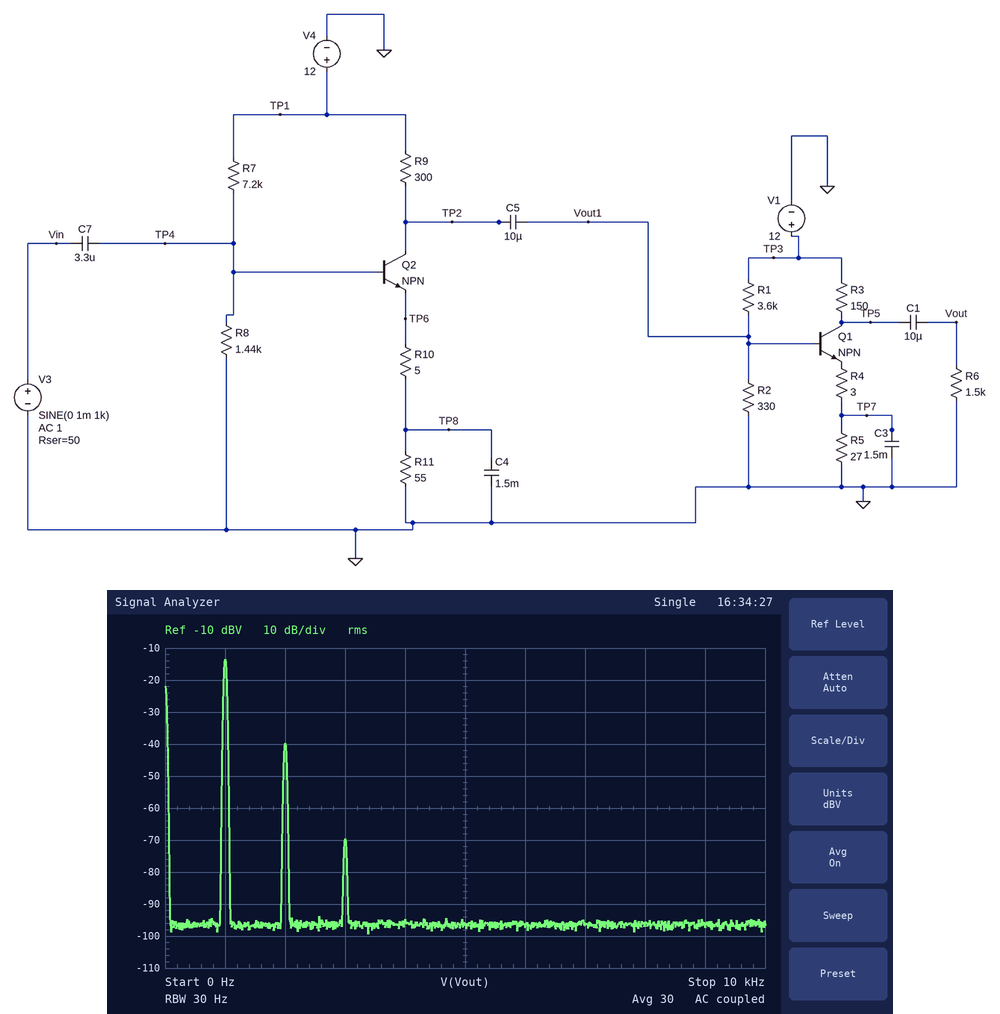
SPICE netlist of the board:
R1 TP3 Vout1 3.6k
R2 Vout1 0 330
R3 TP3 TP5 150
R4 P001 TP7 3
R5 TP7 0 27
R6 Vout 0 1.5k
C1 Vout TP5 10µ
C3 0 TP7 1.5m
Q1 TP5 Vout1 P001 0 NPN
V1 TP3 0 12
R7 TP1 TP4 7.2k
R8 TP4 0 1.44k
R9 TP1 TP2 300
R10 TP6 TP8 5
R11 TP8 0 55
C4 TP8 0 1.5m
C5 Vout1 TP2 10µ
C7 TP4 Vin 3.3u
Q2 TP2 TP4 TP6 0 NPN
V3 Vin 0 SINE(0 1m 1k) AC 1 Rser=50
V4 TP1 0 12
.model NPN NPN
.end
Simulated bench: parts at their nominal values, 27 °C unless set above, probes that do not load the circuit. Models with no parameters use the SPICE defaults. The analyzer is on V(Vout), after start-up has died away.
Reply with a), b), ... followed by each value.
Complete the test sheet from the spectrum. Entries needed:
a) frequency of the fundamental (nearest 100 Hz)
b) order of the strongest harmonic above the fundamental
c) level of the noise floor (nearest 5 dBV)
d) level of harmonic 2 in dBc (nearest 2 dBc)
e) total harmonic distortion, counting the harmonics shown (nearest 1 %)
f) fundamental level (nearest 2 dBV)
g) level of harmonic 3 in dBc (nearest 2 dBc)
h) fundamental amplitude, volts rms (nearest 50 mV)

a) 1.0 kHz
b) 2
c) -95 dBV
d) -26 dBc
e) 5 %
f) -14 dBV
g) -56 dBc
h) 200 mV
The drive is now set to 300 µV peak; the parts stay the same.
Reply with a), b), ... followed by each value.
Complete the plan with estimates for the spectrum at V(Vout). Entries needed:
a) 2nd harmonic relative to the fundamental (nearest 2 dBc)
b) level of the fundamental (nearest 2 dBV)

a) -36 dBc
b) -24 dBV
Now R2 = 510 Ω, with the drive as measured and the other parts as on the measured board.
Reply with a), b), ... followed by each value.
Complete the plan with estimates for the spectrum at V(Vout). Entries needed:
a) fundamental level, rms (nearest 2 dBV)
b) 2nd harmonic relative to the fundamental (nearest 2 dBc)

a) -8 dBV
b) -38 dBc
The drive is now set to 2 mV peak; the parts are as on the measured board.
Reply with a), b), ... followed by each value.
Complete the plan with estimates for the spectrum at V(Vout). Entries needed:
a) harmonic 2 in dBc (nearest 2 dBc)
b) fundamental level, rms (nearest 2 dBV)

a) -20 dBc
b) -8 dBV
